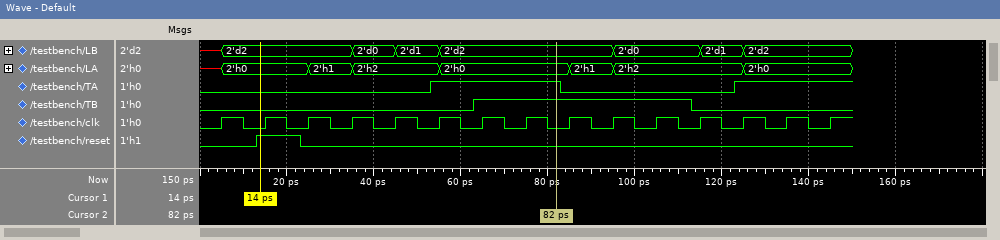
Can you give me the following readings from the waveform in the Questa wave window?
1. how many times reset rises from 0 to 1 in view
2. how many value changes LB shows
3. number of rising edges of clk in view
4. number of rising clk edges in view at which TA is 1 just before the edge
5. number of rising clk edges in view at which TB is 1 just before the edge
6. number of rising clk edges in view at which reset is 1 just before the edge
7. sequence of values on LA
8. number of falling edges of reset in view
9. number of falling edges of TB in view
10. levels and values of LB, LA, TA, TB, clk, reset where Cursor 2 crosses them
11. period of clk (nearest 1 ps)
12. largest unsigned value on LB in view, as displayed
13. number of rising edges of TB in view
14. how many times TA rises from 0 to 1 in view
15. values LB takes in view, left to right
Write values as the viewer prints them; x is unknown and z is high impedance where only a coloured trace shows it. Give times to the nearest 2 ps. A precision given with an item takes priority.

1
7
15
6
5
1
x, 2'h0, 2'h1, 2'h2, 2'h0, 2'h1, 2'h2, 2'h0
1
1
LB=2'd2, LA=2'h0, TA=1, TB=1, clk=0, reset=0
10 ps
2'd2
1
2
x, 2'd2, 2'd0, 2'd1, 2'd2, 2'd0, 2'd1, 2'd2
